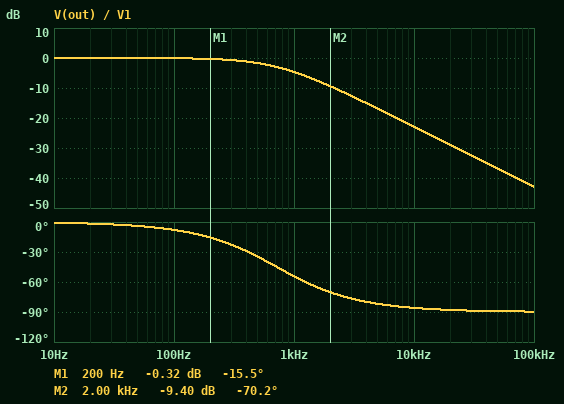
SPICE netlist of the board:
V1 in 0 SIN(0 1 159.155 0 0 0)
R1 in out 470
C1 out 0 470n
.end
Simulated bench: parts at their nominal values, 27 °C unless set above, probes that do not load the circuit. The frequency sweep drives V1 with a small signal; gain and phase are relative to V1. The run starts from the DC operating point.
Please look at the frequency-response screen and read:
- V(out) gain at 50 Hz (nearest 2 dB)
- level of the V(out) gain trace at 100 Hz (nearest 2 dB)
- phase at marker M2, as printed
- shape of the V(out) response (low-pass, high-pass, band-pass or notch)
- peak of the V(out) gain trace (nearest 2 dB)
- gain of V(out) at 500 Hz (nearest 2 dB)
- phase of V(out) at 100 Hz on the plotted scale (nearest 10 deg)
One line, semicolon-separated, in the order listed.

0 dB; 0 dB; -70.2 deg; low-pass; 0 dB; -2 dB; -10 deg
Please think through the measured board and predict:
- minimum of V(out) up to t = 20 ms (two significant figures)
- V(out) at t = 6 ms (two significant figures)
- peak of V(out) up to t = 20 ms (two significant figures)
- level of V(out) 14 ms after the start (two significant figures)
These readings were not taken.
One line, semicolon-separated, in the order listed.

-980 mV; -470 mV; 980 mV; 920 mV
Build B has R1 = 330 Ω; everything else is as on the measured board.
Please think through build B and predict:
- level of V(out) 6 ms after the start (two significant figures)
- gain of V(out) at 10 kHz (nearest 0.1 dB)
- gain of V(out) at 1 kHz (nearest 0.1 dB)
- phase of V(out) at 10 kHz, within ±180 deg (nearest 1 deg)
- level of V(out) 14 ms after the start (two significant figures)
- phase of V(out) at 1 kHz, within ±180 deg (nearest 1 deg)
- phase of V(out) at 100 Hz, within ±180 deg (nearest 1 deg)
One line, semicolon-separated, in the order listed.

-420 mV; -19.8 dB; -2.9 dB; -84 deg; 950 mV; -44 deg; -6 deg
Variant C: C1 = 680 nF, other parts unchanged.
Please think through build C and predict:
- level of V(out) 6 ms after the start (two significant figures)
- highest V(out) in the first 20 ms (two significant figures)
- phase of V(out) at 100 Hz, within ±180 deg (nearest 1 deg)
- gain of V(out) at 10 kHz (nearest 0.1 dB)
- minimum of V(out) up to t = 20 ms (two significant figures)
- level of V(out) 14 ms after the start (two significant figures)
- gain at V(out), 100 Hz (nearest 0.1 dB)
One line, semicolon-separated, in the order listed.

-530 mV; 950 mV; -11 deg; -26.1 dB; -950 mV; 860 mV; -0.2 dB
